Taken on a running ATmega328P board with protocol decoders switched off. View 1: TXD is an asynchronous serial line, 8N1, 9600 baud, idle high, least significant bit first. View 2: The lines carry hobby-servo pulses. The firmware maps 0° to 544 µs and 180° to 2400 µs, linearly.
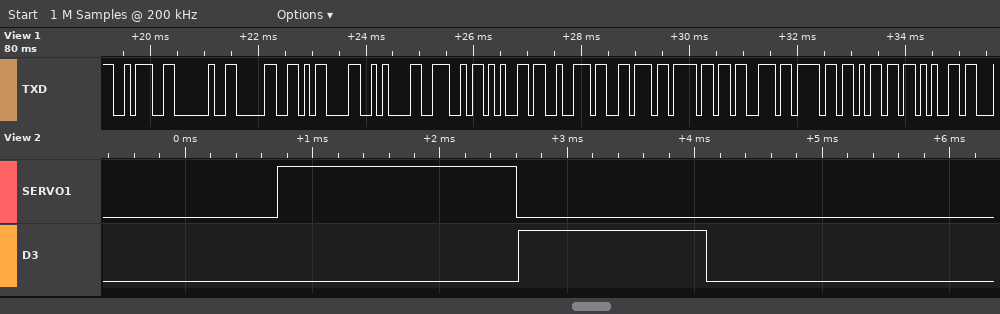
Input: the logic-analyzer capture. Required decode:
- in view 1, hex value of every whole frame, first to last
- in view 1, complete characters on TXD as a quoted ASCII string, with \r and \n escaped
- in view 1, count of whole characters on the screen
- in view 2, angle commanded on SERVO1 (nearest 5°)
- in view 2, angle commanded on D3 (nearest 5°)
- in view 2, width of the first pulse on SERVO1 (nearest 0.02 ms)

3A 20 30 0D 0A 4E 65 72 76 6F 73 6F 6D 65
": 0\r\nNervosome"
14
130°
90°
1.88 ms
